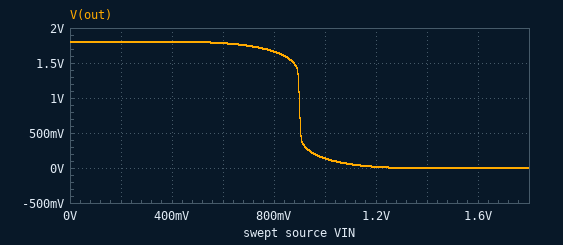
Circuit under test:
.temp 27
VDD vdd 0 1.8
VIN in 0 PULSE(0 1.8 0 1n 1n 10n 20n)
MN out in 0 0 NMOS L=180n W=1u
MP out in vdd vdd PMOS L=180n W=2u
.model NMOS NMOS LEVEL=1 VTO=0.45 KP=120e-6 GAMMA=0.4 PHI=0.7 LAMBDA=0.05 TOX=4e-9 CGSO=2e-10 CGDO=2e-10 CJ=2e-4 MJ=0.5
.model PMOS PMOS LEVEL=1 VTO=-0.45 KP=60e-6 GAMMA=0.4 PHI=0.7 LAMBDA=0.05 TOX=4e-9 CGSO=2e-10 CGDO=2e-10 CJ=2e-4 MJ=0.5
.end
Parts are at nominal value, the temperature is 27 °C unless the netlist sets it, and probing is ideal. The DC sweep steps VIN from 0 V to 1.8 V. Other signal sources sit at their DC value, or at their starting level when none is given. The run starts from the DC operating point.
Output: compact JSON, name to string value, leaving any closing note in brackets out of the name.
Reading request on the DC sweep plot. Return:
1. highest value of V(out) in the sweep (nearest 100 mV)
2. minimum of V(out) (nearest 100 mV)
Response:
{"highest value of V(out) in the sweep": "1.8 V", "minimum of V(out)": "0 V"}
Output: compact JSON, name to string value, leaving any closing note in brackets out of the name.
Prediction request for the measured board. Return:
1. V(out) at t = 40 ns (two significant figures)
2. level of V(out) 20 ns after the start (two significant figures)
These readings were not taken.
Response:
{"V(out) at t = 40 ns": "1.8 V", "level of V(out) 20 ns after the start": "1.8 V"}
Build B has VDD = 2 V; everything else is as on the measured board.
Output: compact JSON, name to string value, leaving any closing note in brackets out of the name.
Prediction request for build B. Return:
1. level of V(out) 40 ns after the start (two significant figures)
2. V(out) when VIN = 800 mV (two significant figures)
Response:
{"level of V(out) 40 ns after the start": "2.0 V", "V(out) when VIN = 800 mV": "1.9 V"}
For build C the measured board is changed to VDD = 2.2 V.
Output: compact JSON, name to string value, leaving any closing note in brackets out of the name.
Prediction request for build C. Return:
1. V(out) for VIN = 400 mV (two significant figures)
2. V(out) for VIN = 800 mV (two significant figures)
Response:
{"V(out) for VIN = 400 mV": "2.2 V", "V(out) for VIN = 800 mV": "2.1 V"}
